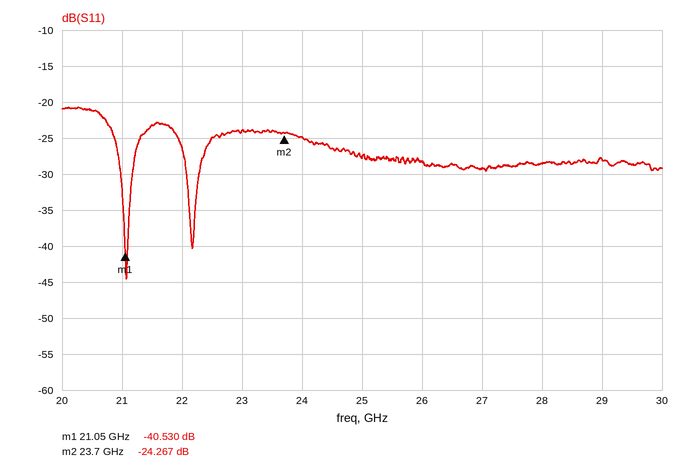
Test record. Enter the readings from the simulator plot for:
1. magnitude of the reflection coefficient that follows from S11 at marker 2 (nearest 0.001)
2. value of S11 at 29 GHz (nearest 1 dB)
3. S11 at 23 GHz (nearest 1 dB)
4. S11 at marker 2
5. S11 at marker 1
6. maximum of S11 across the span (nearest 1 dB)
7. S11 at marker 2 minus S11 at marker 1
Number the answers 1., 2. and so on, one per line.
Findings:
1. 0.061
2. -28 dB
3. -24 dB
4. -24.267 dB
5. -40.530 dB
6. -21 dB
7. 16.263 dB
